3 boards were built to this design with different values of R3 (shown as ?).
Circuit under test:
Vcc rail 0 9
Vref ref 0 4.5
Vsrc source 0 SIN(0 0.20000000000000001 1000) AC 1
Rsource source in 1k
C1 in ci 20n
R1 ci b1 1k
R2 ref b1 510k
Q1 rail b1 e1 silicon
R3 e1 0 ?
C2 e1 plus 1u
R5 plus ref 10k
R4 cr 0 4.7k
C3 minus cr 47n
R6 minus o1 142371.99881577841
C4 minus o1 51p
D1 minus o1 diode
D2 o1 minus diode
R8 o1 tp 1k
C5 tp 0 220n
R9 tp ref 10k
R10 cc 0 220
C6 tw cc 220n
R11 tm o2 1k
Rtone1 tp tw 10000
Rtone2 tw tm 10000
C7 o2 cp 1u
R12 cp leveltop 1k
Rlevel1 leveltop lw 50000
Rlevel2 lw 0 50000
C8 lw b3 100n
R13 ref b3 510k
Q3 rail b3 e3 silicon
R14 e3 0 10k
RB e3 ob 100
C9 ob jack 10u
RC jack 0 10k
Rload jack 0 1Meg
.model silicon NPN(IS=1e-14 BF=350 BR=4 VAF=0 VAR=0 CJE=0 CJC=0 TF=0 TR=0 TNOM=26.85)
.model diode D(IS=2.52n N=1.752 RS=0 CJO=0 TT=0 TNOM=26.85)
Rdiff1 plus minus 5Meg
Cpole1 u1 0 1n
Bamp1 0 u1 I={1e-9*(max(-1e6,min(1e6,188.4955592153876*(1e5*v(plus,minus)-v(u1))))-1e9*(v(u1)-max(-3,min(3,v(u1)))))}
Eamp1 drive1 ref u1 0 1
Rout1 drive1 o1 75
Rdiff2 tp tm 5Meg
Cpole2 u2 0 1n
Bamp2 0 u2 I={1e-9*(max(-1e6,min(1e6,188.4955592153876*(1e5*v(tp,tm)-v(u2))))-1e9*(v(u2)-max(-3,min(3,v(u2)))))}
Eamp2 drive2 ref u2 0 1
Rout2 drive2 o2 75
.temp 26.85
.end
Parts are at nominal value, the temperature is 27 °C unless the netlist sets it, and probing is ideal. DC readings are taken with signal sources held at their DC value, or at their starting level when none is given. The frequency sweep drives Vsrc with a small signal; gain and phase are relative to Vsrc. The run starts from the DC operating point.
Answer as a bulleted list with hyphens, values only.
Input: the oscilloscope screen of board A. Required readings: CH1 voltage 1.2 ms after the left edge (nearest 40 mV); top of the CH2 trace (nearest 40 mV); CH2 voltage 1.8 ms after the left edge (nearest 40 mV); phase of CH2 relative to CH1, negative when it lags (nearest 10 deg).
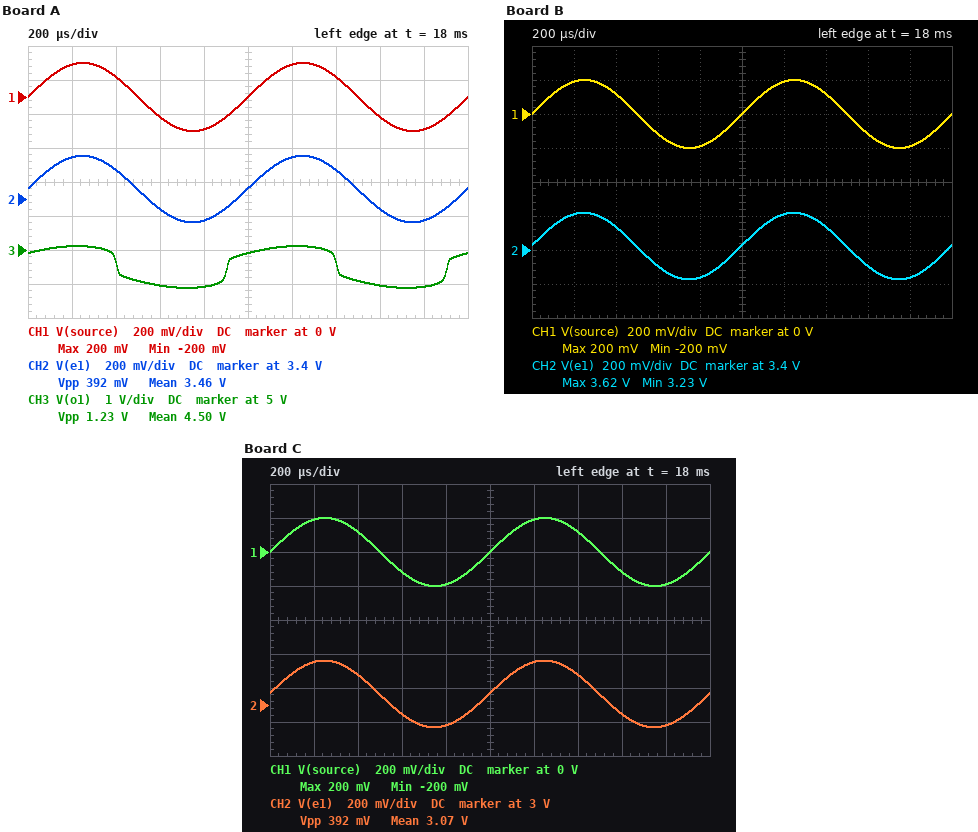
- 200 mV
- 3.64 V
- 3.28 V
- 0 deg
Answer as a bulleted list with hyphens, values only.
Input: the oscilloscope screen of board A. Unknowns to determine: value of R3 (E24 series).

- 12 kΩ
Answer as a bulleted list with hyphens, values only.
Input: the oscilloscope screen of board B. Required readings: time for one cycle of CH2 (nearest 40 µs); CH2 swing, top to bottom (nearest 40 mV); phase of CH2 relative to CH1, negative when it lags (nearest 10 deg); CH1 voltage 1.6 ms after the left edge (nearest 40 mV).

- 1.00 ms
- 400 mV
- 0 deg
- -120 mV
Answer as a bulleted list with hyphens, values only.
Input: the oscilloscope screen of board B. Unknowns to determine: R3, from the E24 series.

- 11 kΩ
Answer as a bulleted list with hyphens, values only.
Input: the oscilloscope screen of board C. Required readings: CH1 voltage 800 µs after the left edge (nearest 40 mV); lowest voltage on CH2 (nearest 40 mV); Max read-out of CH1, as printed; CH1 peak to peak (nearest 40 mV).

- -200 mV
- 2.88 V
- 200 mV
- 400 mV
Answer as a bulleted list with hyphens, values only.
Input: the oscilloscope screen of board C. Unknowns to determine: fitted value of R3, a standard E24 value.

- 5.6 kΩ
